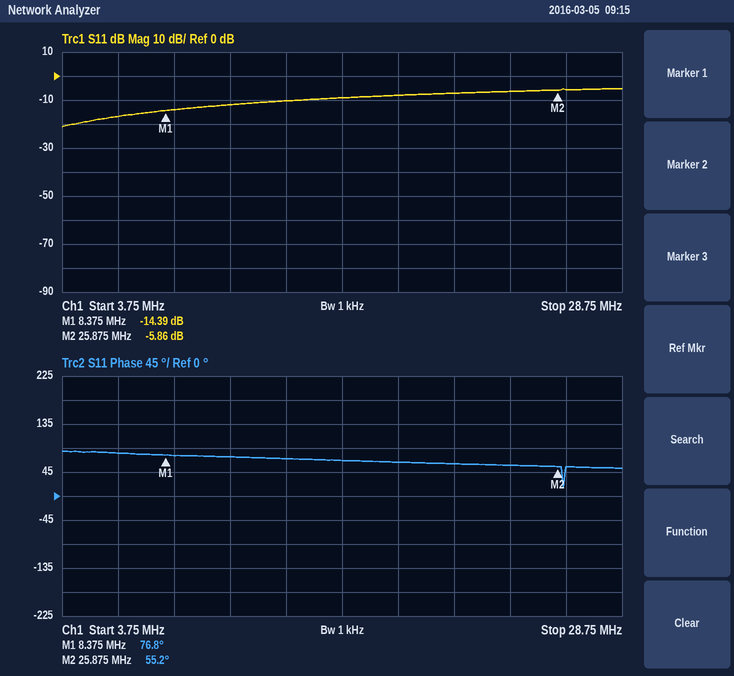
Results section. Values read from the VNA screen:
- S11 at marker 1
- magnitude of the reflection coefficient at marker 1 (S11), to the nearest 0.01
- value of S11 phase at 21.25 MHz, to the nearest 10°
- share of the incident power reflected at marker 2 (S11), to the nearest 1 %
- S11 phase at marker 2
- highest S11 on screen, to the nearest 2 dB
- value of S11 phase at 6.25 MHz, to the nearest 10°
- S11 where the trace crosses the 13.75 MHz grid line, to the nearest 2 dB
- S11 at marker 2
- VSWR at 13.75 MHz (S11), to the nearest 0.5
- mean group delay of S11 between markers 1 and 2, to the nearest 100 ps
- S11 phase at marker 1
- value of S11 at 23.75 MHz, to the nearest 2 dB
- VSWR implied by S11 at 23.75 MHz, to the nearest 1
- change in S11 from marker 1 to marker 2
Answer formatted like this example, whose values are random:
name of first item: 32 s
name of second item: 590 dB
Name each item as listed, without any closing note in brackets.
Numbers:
S11 at marker 1: -14.39 dB
magnitude of the reflection coefficient at marker 1 (S11), to the nearest 0.01: 0.19
value of S11 phase at 21.25 MHz, to the nearest 10°: 60°
share of the incident power reflected at marker 2 (S11), to the nearest 1 %: 26 %
S11 phase at marker 2: 55.2°
highest S11 on screen, to the nearest 2 dB: -6 dB
value of S11 phase at 6.25 MHz, to the nearest 10°: 80°
S11 where the trace crosses the 13.75 MHz grid line, to the nearest 2 dB: -10 dB
S11 at marker 2: -5.86 dB
VSWR at 13.75 MHz (S11), to the nearest 0.5: 2.0
mean group delay of S11 between markers 1 and 2, to the nearest 100 ps: 3.4 ns
S11 phase at marker 1: 76.8°
value of S11 at 23.75 MHz, to the nearest 2 dB: -6 dB
VSWR implied by S11 at 23.75 MHz, to the nearest 1: 3
change in S11 from marker 1 to marker 2: 8.53 dB
